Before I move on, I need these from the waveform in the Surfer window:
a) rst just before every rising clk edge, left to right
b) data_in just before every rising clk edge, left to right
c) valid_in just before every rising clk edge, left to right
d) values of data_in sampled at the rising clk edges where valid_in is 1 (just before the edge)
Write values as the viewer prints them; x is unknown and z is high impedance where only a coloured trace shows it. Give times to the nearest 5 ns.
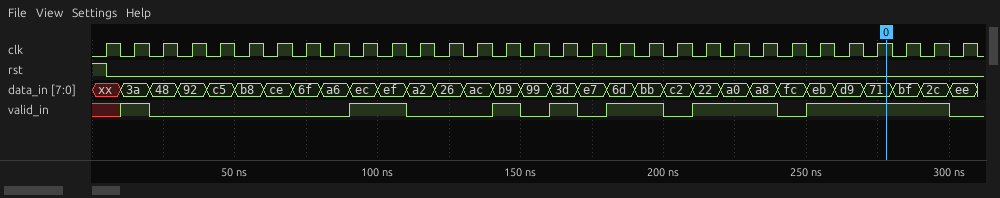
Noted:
1 0 0 0 0 0 0 0 0 0 0 0 0 0 0 0 0 0 0 0 0 0 0 0 0 0 0 0 0 0 0
xx, 3a, 48, 92, c5, b8, ce, 6f, a6, ec, ef, a2, 26, ac, b9, 99, 3d, e7, 6d, bb, c2, 22, a0, a8, fc, eb, d9, 71, bf, 2c, ee
x 1 0 0 0 0 0 0 0 1 1 0 0 0 1 0 1 0 1 1 0 1 1 1 0 1 1 1 1 1 0
3a, ec, ef, b9, 3d, 6d, bb, 22, a0, a8, eb, d9, 71, bf, 2c
